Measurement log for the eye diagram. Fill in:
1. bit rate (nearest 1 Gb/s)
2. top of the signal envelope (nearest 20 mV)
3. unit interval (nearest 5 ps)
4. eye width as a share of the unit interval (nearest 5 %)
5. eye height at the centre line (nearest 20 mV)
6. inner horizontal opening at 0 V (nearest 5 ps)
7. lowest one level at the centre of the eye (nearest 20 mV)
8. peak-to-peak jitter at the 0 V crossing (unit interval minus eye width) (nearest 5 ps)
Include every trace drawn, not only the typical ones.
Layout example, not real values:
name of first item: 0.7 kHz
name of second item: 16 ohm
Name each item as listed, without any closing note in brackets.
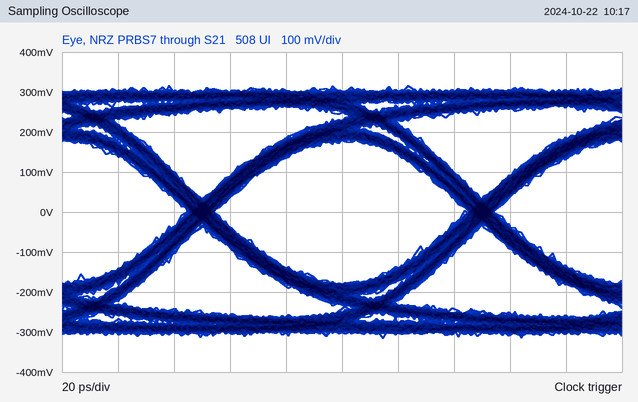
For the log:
bit rate: 10 Gb/s
top of the signal envelope: 320 mV
unit interval: 100 ps
eye width as a share of the unit interval: 90 %
eye height at the centre line: 360 mV
inner horizontal opening at 0 V: 90 ps
lowest one level at the centre of the eye: 180 mV
peak-to-peak jitter at the 0 V crossing (unit interval minus eye width): 10 ps
